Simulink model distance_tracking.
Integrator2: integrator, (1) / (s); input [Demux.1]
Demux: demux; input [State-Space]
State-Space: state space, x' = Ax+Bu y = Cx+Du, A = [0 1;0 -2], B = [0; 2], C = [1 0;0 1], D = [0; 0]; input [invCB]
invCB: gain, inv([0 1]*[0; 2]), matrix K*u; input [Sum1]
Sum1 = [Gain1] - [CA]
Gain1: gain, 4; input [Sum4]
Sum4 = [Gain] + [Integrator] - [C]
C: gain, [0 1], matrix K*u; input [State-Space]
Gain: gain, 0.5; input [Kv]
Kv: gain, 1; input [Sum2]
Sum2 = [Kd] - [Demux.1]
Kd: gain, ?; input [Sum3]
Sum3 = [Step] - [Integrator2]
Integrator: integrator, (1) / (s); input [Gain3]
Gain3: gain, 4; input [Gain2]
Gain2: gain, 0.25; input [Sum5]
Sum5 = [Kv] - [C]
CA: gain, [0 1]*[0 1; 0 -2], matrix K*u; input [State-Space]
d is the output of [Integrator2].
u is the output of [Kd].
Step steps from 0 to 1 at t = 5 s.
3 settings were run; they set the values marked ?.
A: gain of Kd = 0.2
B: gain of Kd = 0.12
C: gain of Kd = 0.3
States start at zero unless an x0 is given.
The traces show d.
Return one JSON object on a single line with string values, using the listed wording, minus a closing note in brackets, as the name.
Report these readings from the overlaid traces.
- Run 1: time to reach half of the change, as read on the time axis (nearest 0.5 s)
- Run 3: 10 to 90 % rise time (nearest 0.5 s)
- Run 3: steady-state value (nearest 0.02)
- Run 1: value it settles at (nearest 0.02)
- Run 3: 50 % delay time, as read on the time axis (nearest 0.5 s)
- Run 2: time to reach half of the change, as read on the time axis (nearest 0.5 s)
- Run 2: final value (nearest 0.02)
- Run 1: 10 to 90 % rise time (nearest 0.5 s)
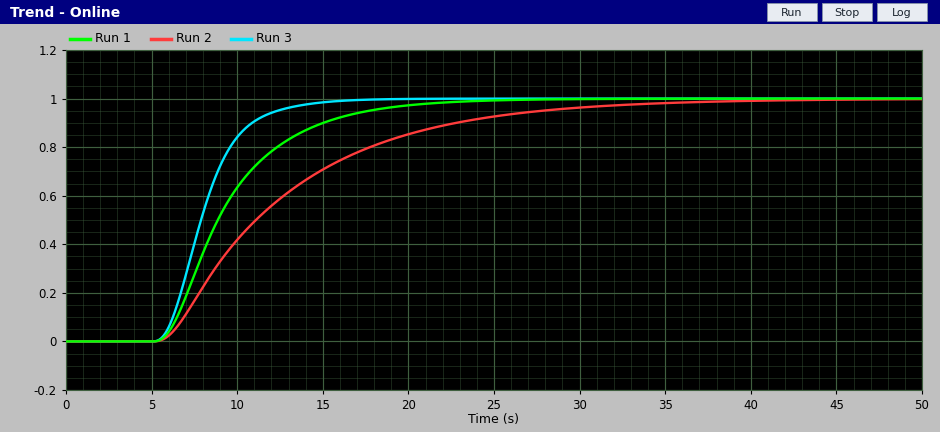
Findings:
{"Run 1: time to reach half of the change, as read on the time axis": "9.0 s", "Run 3: 10 to 90 % rise time": "4.5 s", "Run 3: steady-state value": "1.00", "Run 1: value it settles at": "1.00", "Run 3: 50 % delay time, as read on the time axis": "8.0 s", "Run 2: time to reach half of the change, as read on the time axis": "11.0 s", "Run 2: final value": "1.00", "Run 1: 10 to 90 % rise time": "8.5 s"}
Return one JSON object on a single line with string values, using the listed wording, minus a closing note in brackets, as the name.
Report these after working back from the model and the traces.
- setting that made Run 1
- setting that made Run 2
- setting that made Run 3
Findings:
{"setting that made Run 1": "A", "setting that made Run 2": "B", "setting that made Run 3": "C"}
